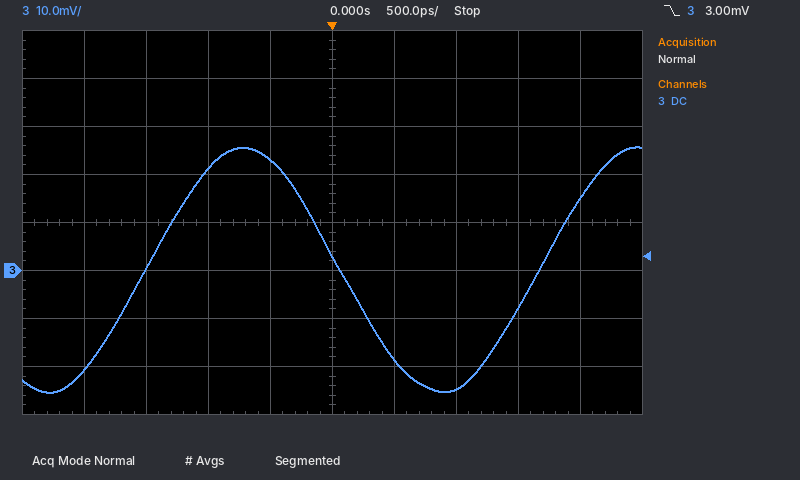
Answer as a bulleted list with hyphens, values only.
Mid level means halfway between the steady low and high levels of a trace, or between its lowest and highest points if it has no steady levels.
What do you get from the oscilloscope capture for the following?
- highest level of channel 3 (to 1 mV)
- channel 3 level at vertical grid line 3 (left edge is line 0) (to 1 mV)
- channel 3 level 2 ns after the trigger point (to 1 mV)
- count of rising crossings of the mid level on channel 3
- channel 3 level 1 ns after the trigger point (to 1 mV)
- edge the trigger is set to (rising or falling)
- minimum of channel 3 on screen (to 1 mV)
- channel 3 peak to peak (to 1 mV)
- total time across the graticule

- 26 mV
- 21 mV
- 15 mV
- 2
- -25 mV
- falling
- -25 mV
- 51 mV
- 5 ns
